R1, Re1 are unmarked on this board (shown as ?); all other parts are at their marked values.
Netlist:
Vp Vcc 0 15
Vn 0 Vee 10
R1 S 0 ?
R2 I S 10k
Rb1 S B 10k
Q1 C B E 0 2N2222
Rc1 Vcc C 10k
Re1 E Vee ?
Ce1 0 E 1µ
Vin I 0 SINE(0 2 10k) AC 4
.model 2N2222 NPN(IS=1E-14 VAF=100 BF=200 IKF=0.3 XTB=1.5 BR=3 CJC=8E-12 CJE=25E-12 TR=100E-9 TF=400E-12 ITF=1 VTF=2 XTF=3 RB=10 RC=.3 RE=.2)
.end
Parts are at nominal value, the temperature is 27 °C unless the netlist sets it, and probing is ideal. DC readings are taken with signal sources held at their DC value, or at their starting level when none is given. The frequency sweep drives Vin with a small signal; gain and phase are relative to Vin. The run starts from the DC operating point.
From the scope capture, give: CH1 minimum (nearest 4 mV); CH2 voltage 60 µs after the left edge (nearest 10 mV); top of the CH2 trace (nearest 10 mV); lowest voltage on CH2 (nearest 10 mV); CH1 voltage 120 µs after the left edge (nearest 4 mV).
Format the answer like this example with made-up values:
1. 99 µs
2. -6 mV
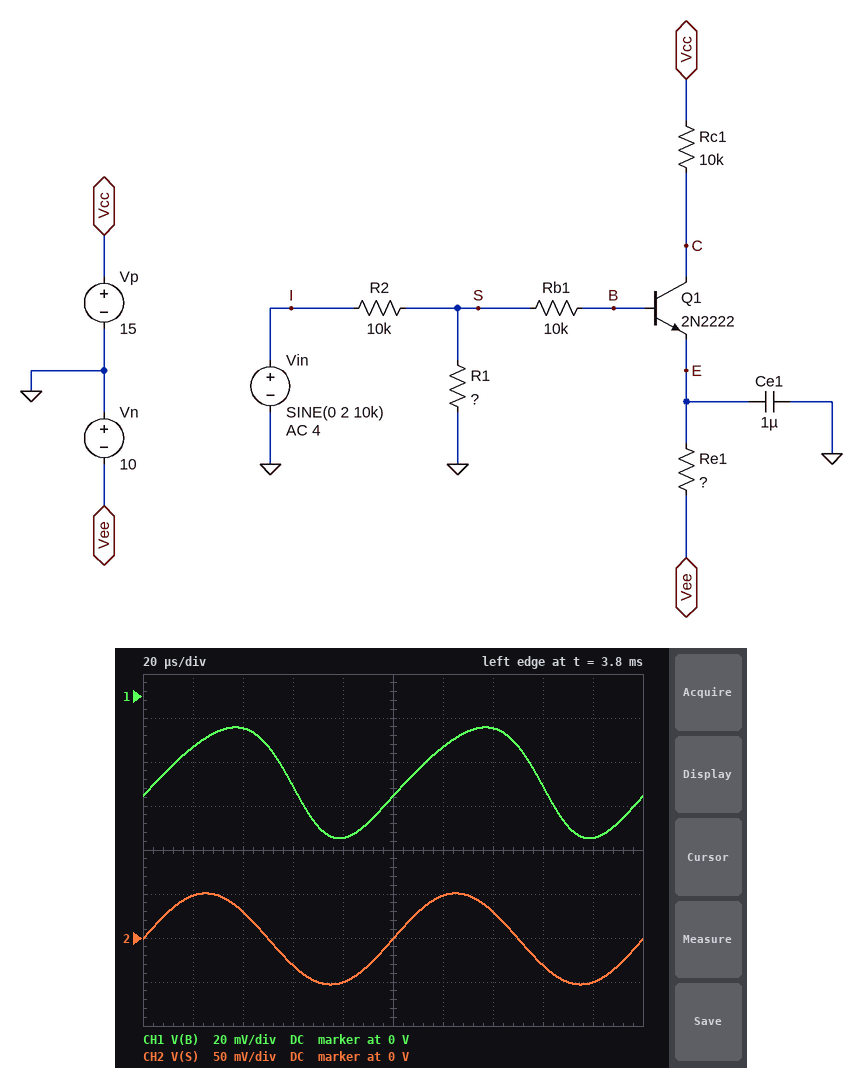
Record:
1. -64 mV
2. -30 mV
3. 50 mV
4. -50 mV
5. -24 mV
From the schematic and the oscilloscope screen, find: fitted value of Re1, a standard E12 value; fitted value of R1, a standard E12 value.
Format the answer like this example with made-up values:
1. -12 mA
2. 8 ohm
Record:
1. 12 kΩ
2. 270 Ω
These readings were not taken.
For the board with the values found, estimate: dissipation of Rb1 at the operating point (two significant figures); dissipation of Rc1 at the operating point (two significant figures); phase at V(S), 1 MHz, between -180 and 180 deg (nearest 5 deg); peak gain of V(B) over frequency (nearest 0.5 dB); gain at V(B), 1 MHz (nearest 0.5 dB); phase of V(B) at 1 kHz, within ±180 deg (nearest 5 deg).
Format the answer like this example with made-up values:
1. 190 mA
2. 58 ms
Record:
1. 130 nW
2. 6.0 mW
3. 0 deg
4. -31.5 dB
5. -68.0 dB
6. -15 deg
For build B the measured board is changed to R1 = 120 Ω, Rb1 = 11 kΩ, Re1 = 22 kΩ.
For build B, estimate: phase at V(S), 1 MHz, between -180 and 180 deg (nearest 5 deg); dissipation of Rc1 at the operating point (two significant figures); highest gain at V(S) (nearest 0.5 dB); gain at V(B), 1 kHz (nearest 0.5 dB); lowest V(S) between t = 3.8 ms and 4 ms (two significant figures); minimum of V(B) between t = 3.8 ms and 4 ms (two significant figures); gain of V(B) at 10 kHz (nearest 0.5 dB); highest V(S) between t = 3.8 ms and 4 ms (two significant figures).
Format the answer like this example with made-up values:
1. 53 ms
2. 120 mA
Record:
1. 0 deg
2. 1.8 mW
3. -38.5 dB
4. -39.5 dB
5. -24 mV
6. -36 mV
7. -43.5 dB
8. 23 mV
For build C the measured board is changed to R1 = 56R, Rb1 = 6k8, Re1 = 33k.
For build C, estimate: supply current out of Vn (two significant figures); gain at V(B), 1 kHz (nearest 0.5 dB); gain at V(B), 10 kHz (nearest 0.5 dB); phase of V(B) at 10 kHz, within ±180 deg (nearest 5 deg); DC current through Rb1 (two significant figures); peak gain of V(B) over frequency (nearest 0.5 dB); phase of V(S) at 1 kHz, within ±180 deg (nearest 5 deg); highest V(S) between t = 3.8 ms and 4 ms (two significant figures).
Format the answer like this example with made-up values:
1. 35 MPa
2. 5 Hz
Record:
1. 280 µA
2. -46.0 dB
3. -47.5 dB
4. -10 deg
5. 1.3 µA
6. -45.0 dB
7. 0 deg
8. 11 mV
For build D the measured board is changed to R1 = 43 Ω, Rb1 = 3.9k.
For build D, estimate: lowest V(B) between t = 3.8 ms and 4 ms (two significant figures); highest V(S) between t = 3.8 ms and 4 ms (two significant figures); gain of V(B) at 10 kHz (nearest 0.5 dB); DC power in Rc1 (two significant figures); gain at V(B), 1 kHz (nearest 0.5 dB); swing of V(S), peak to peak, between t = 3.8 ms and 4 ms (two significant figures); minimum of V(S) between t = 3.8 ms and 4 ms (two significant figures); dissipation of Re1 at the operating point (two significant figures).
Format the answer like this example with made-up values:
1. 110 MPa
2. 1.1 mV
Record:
1. -20 mV
2. 8.4 mV
3. -50.5 dB
4. 6.0 mW
5. -47.5 dB
6. 17 mV
7. -8.7 mV
8. 7.3 mW
